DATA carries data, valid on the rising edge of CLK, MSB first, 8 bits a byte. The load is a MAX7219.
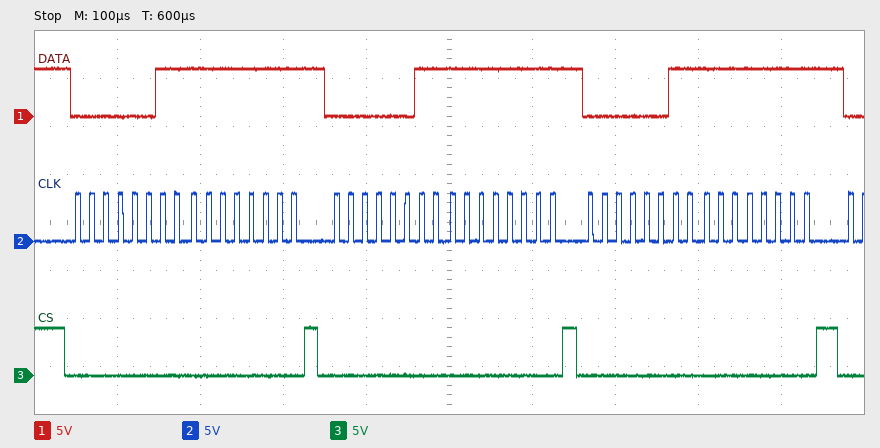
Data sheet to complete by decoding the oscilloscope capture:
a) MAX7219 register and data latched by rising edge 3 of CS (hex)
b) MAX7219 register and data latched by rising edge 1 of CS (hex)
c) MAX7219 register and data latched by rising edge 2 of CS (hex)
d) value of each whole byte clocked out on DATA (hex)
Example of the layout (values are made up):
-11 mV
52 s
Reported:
register 0x3, data 0xFF
register 0x3, data 0xFF
register 0x3, data 0xFF
0x03 0xFF 0x03 0xFF 0x03 0xFF
